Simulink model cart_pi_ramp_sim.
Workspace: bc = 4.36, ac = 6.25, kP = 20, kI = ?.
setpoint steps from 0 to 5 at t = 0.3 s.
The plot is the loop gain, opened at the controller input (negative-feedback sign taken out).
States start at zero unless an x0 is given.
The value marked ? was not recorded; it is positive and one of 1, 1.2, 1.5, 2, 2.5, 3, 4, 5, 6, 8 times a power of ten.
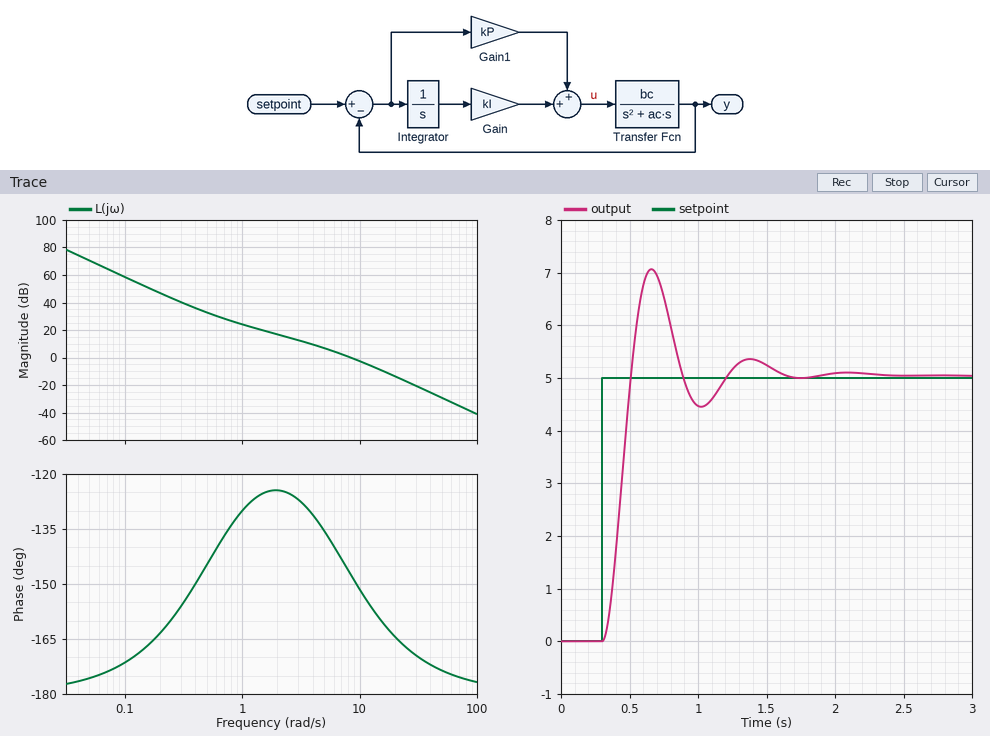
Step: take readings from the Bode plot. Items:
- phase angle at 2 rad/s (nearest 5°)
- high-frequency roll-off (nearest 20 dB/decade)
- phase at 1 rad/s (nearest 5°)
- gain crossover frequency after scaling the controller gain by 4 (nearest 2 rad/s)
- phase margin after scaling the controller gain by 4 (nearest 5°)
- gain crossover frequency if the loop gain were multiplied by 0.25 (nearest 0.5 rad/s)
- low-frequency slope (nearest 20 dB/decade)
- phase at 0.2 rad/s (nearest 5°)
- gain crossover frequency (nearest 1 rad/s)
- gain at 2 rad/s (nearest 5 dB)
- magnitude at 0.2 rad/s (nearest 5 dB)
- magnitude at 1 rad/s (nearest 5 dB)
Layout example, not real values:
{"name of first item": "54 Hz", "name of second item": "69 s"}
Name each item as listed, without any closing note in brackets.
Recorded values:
{"phase angle at 2 rad/s": "-125°", "high-frequency roll-off": "-40 dB/decade", "phase at 1 rad/s": "-130°", "gain crossover frequency after scaling the controller gain by 4": "18 rad/s", "phase margin after scaling the controller gain by 4": "15°", "gain crossover frequency if the loop gain were multiplied by 0.25": "3.0 rad/s", "low-frequency slope": "-40 dB/decade", "phase at 0.2 rad/s": "-165°", "gain crossover frequency": "8 rad/s", "gain at 2 rad/s": "15 dB", "magnitude at 0.2 rad/s": "45 dB", "magnitude at 1 rad/s": "25 dB"}
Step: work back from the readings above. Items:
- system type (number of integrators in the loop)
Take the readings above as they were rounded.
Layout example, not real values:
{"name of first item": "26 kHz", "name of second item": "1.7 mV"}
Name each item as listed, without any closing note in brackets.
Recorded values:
{"system type": "2"}
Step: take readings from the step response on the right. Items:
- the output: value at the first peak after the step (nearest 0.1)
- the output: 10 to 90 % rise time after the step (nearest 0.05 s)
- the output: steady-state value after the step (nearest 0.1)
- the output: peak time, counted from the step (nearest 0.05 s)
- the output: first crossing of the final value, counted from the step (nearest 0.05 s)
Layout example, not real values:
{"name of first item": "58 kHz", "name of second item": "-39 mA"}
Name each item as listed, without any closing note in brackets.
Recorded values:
{"the output: value at the first peak after the step": "7.1", "the output: 10 to 90 % rise time after the step": "0.15 s", "the output: steady-state value after the step": "5.0", "the output: peak time, counted from the step": "0.35 s", "the output: first crossing of the final value, counted from the step": "0.20 s"}
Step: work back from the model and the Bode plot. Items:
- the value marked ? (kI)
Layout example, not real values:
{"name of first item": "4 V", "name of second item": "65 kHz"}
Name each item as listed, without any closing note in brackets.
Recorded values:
{"the value marked ?": "12"}
